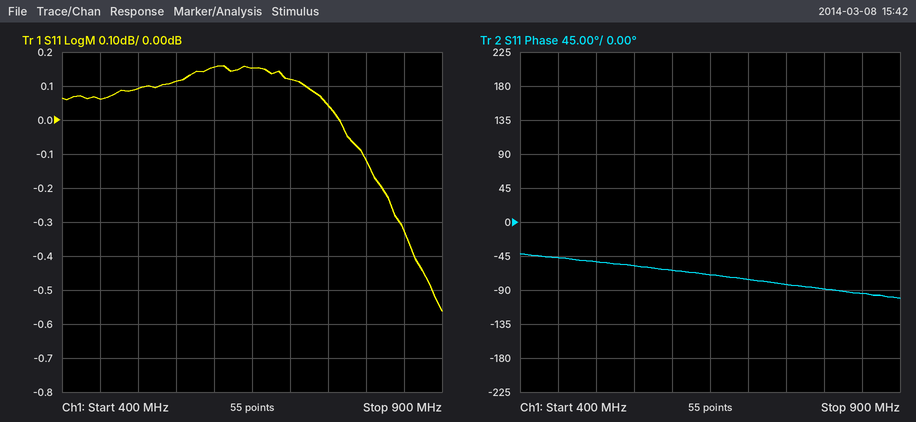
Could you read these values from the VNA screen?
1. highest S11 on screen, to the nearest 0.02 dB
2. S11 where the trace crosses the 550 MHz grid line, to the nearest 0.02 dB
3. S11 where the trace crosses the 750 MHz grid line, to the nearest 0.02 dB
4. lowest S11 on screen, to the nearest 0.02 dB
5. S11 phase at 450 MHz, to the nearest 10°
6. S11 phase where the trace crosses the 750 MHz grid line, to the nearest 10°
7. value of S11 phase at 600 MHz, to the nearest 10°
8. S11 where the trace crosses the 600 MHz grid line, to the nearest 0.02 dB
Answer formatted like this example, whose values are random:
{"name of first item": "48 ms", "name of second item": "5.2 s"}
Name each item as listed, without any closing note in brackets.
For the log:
{"highest S11 on screen, to the nearest 0.02 dB": "0.16 dB", "S11 where the trace crosses the 550 MHz grid line, to the nearest 0.02 dB": "0.12 dB", "S11 where the trace crosses the 750 MHz grid line, to the nearest 0.02 dB": "0.04 dB", "lowest S11 on screen, to the nearest 0.02 dB": "-0.56 dB", "S11 phase at 450 MHz, to the nearest 10°": "-50°", "S11 phase where the trace crosses the 750 MHz grid line, to the nearest 10°": "-80°", "value of S11 phase at 600 MHz, to the nearest 10°": "-60°", "S11 where the trace crosses the 600 MHz grid line, to the nearest 0.02 dB": "0.16 dB"}
